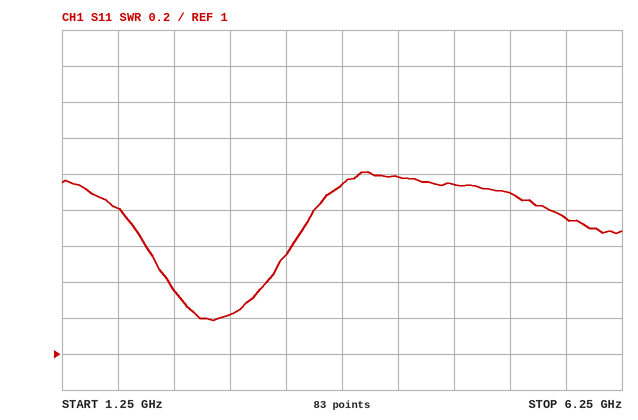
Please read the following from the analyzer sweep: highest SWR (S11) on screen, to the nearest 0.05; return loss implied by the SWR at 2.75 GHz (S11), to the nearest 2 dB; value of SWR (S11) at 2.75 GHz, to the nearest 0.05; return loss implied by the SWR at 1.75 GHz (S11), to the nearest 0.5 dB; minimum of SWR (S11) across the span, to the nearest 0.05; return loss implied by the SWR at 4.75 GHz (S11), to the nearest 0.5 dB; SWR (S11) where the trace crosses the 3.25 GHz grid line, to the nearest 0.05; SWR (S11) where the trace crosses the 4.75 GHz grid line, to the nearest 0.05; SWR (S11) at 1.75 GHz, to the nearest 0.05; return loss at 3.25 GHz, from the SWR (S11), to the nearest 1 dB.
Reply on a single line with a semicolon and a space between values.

2.00; 20 dB; 1.20; 11.0 dB; 1.20; 10.0 dB; 1.55; 1.95; 1.80; 13 dB
